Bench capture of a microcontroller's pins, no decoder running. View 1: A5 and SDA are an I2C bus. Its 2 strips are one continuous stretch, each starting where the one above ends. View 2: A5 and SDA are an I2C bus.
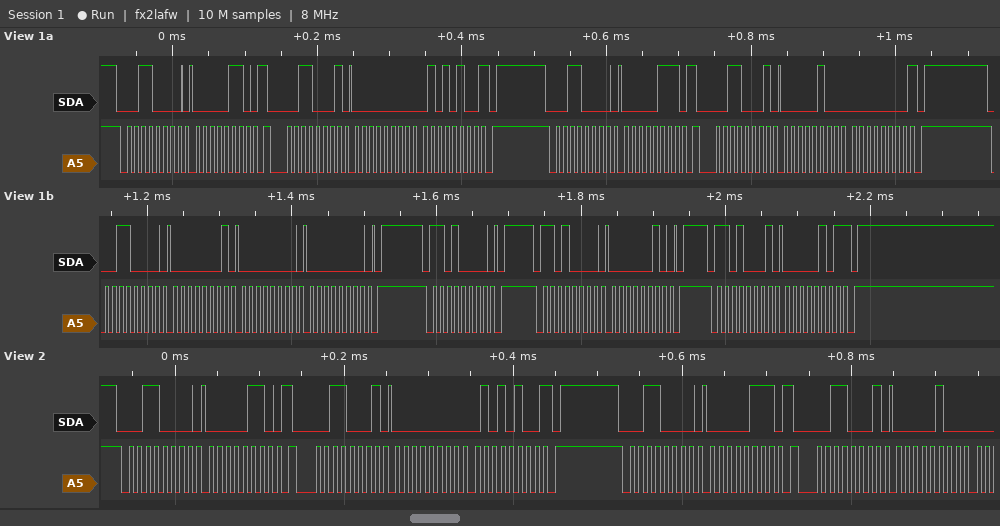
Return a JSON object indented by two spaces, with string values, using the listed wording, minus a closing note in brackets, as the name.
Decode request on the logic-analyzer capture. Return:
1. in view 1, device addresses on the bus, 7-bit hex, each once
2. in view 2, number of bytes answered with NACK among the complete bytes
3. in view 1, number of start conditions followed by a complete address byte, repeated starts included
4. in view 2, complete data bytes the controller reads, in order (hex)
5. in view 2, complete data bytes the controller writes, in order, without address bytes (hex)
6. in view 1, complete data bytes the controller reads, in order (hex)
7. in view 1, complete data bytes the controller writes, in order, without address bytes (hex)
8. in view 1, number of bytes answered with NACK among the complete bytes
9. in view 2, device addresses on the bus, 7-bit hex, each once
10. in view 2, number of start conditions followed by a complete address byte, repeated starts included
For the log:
{
  "in view 1, device addresses on the bus, 7-bit hex, each once": "0x18 0x68",
  "in view 2, number of bytes answered with NACK among the complete bytes": "1",
  "in view 1, number of start conditions followed by a complete address byte, repeated starts included": "8",
  "in view 2, complete data bytes the controller reads, in order": "00 54 04",
  "in view 2, complete data bytes the controller writes, in order, without address bytes": "06 07",
  "in view 1, complete data bytes the controller reads, in order": "00 54 04 00 05",
  "in view 1, complete data bytes the controller writes, in order, without address bytes": "06 07 01 00 00 02",
  "in view 1, number of bytes answered with NACK among the complete bytes": "3",
  "in view 2, device addresses on the bus, 7-bit hex, each once": "0x18",
  "in view 2, number of start conditions followed by a complete address byte, repeated starts included": "4"
}
